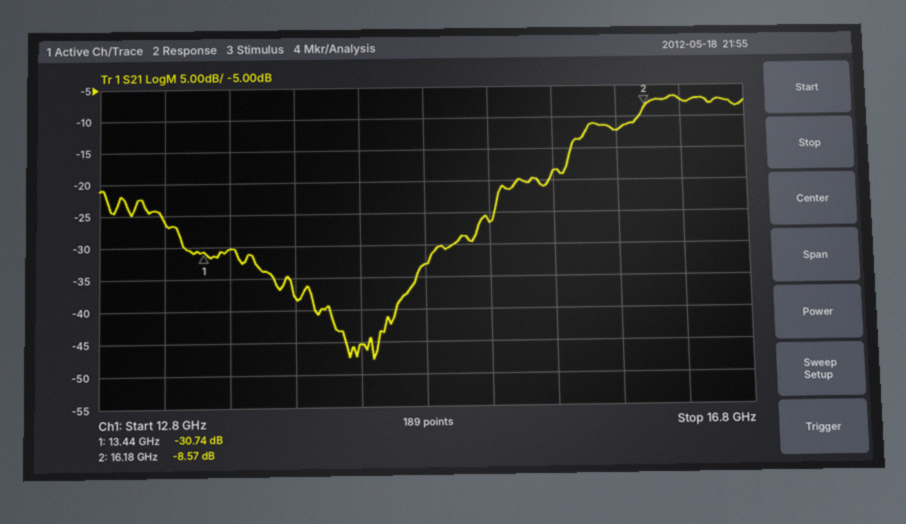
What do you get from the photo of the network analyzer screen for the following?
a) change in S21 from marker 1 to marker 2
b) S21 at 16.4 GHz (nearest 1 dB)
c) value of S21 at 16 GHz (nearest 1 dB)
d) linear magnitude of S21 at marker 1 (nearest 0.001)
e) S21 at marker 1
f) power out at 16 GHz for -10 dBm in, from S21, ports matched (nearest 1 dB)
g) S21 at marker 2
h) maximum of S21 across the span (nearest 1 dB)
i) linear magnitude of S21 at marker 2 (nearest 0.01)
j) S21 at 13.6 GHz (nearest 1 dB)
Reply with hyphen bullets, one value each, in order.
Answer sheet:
- 22.17 dB
- -7 dB
- -12 dB
- 0.029
- -30.74 dB
- -22 dBm
- -8.57 dB
- -7 dB
- 0.37
- -30 dB
